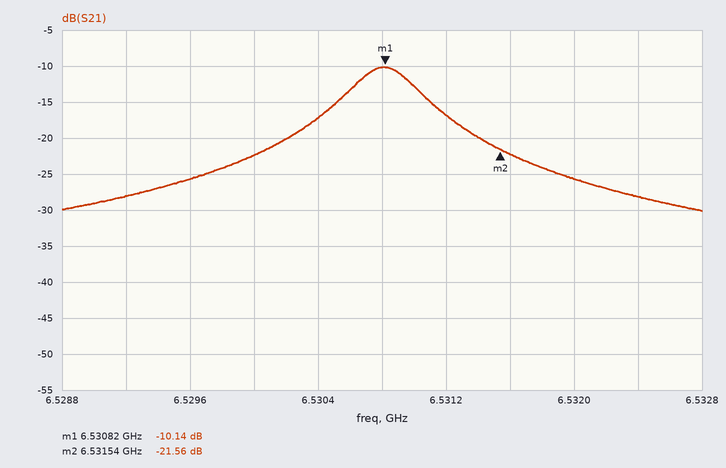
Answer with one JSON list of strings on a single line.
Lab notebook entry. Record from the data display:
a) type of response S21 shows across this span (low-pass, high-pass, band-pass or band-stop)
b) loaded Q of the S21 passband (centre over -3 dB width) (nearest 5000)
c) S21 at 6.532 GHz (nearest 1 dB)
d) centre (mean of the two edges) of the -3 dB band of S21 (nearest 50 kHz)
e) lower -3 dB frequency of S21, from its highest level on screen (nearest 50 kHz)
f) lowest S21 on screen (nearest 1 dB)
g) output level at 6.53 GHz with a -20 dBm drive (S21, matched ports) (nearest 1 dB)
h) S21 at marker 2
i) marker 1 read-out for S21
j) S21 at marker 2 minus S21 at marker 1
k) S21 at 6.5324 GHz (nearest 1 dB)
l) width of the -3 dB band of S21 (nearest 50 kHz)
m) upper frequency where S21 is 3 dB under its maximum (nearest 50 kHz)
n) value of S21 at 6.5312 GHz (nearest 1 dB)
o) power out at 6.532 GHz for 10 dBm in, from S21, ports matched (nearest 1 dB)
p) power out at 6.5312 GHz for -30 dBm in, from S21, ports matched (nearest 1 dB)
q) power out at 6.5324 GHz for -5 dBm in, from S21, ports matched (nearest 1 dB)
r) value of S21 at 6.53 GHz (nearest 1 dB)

["band-pass", "15000", "-26 dB", "6.53080 GHz", "6.53060 GHz", "-30 dB", "-42 dBm", "-21.56 dB", "-10.14 dB", "-11.42 dB", "-28 dB", "400 kHz", "6.53100 GHz", "-17 dB", "-16 dBm", "-47 dBm", "-33 dBm", "-22 dB"]
